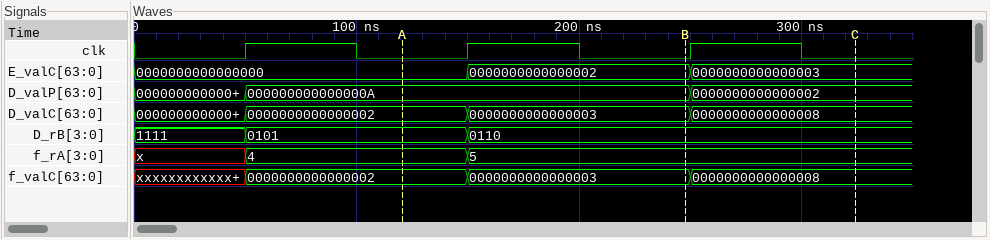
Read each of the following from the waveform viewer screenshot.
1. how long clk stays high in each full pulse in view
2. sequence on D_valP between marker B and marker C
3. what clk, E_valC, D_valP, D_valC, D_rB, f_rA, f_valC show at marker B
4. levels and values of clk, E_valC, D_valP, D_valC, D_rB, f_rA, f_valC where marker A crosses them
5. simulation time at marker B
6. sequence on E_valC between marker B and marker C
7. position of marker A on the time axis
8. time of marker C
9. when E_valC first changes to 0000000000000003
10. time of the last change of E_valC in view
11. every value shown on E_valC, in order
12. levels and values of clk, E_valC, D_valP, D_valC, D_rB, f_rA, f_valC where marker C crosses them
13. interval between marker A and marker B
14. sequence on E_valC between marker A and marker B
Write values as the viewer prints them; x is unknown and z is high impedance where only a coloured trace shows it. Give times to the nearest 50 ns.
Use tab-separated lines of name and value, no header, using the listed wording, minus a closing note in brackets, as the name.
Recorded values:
how long clk stays high in each full pulse in view	50 ns, 50 ns, 50 ns
sequence on D_valP between marker B and marker C	000000000000000A, 0000000000000002
what clk, E_valC, D_valP, D_valC, D_rB, f_rA, f_valC show at marker B	clk=0, E_valC=0000000000000002, D_valP=000000000000000A, D_valC=0000000000000003, D_rB=0110, f_rA=5, f_valC=0000000000000003
levels and values of clk, E_valC, D_valP, D_valC, D_rB, f_rA, f_valC where marker A crosses them	clk=0, E_valC=0000000000000000, D_valP=000000000000000A, D_valC=0000000000000002, D_rB=0101, f_rA=4, f_valC=0000000000000002
simulation time at marker B	250 ns
sequence on E_valC between marker B and marker C	0000000000000002, 0000000000000003
position of marker A on the time axis	100 ns
time of marker C	300 ns
when E_valC first changes to 0000000000000003	250 ns
time of the last change of E_valC in view	250 ns
every value shown on E_valC, in order	0000000000000000, 0000000000000002, 0000000000000003
levels and values of clk, E_valC, D_valP, D_valC, D_rB, f_rA, f_valC where marker C crosses them	clk=0, E_valC=0000000000000003, D_valP=0000000000000002, D_valC=0000000000000008, D_rB=0110, f_rA=5, f_valC=0000000000000008
interval between marker A and marker B	150 ns
sequence on E_valC between marker A and marker B	0000000000000000, 0000000000000002
